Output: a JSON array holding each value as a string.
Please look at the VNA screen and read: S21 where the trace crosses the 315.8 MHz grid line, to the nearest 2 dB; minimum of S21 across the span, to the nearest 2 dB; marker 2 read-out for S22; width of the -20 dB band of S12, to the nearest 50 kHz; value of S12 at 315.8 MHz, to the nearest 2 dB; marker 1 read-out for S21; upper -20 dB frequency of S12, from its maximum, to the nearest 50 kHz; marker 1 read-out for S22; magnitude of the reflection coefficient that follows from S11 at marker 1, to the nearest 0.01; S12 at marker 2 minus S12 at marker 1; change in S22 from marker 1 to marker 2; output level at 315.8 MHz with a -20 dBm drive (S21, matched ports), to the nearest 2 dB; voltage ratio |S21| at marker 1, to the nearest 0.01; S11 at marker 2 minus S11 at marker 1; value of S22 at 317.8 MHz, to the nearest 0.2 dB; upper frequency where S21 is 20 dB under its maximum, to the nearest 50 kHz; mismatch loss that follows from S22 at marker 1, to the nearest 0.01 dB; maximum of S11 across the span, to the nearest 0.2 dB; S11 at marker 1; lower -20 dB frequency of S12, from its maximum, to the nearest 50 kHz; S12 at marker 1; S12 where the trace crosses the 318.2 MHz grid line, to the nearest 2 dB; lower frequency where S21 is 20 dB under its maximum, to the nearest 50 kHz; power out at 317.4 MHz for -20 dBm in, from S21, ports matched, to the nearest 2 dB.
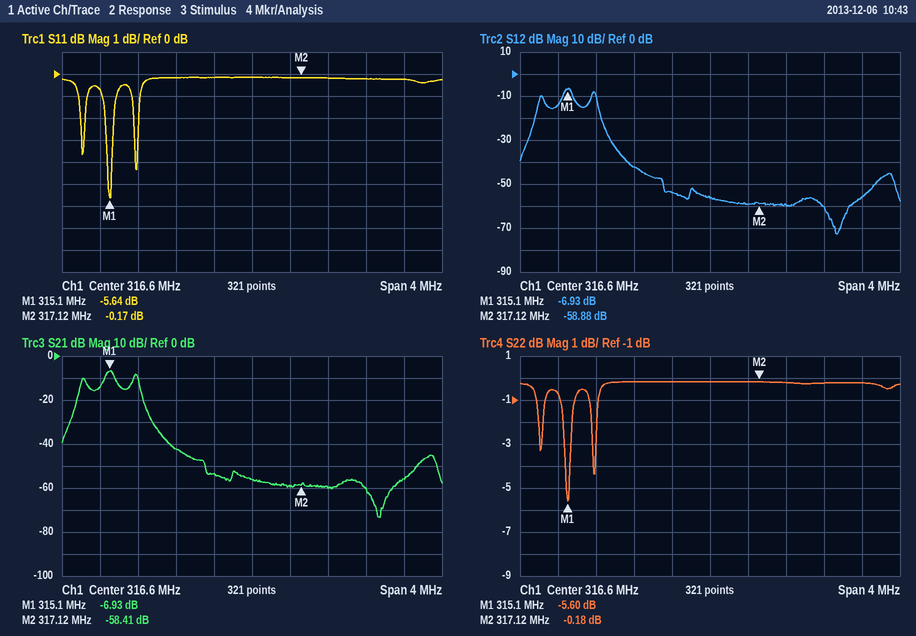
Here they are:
["-42 dB", "-74 dB", "-0.18 dB", "800 kHz", "-42 dB", "-6.93 dB", "315.50 MHz", "-5.60 dB", "0.52", "-51.95 dB", "5.42 dB", "-62 dBm", "0.45", "5.47 dB", "-0.2 dB", "315.50 MHz", "1.40 dB", "-0.2 dB", "-5.64 dB", "314.70 MHz", "-6.93 dB", "-56 dB", "314.70 MHz", "-80 dBm"]
